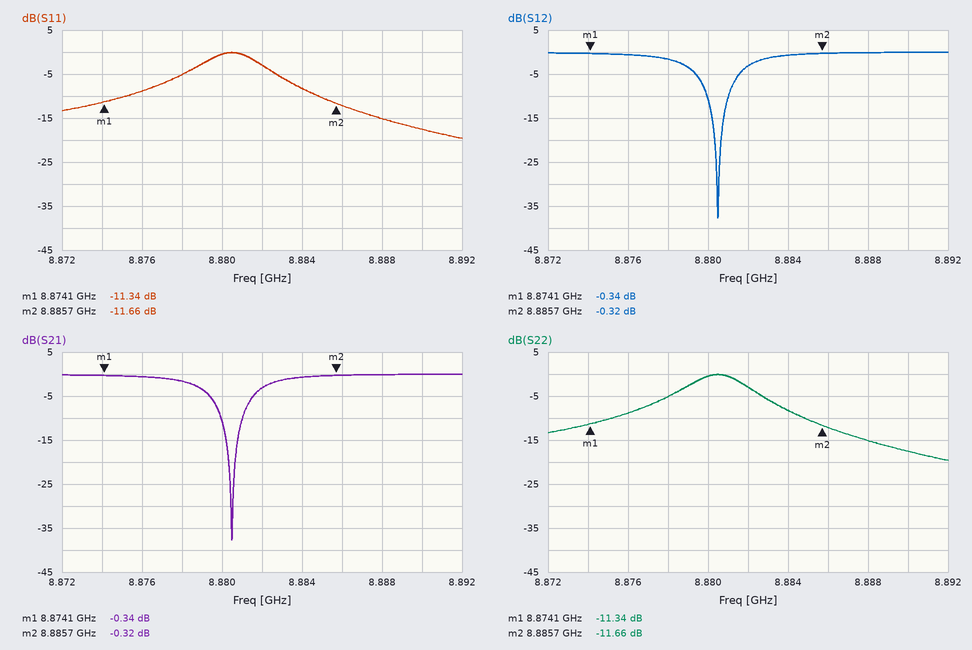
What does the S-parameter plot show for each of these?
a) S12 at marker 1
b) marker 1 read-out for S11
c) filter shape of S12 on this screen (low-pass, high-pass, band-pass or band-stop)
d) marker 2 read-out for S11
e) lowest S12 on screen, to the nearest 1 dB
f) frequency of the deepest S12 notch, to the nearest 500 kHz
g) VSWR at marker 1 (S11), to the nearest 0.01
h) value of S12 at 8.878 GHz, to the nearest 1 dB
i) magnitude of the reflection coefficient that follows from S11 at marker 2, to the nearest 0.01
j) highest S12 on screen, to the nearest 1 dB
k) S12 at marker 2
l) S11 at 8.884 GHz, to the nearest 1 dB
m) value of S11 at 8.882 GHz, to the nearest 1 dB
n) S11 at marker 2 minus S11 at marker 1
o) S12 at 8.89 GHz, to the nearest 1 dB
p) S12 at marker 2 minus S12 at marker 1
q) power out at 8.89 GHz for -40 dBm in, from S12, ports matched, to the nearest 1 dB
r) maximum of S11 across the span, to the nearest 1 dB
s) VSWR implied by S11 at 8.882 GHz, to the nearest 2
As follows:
-0.34 dB
-11.34 dB
band-stop
-11.66 dB
-38 dB
8.8805 GHz
1.74
-2 dB
0.26
0 dB
-0.32 dB
-8 dB
-3 dB
-0.32 dB
0 dB
0.02 dB
-40 dBm
0 dB
6
